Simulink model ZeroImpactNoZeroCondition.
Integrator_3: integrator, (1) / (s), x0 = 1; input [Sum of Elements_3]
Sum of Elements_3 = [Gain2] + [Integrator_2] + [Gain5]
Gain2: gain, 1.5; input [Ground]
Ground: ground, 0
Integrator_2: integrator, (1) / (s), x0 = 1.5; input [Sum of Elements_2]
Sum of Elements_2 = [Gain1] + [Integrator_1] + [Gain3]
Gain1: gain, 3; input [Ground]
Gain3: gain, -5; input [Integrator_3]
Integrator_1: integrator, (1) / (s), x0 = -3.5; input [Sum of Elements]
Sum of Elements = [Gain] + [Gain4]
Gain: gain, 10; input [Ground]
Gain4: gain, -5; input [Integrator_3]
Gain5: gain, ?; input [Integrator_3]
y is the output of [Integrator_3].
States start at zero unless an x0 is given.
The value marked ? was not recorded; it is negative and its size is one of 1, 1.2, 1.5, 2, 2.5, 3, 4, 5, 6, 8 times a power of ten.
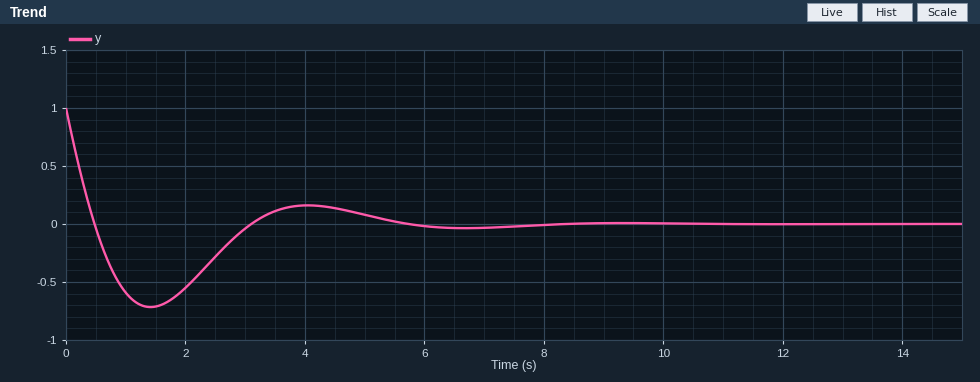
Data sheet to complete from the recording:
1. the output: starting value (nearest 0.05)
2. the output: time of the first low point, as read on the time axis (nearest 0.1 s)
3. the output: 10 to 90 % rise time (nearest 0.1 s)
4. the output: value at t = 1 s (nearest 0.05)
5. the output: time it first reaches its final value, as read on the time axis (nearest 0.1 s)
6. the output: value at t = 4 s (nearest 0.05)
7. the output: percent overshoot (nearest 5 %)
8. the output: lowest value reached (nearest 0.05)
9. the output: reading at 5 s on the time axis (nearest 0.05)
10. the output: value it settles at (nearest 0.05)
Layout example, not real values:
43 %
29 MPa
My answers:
1.00
1.4 s
0.4 s
-0.60
0.5 s
0.15
70 %
-0.70
0.10
0.00
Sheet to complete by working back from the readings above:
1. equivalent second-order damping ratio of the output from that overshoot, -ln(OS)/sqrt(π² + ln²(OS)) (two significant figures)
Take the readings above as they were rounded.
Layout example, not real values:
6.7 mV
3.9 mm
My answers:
0.11
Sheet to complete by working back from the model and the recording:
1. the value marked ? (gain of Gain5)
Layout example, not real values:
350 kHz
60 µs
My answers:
-4
